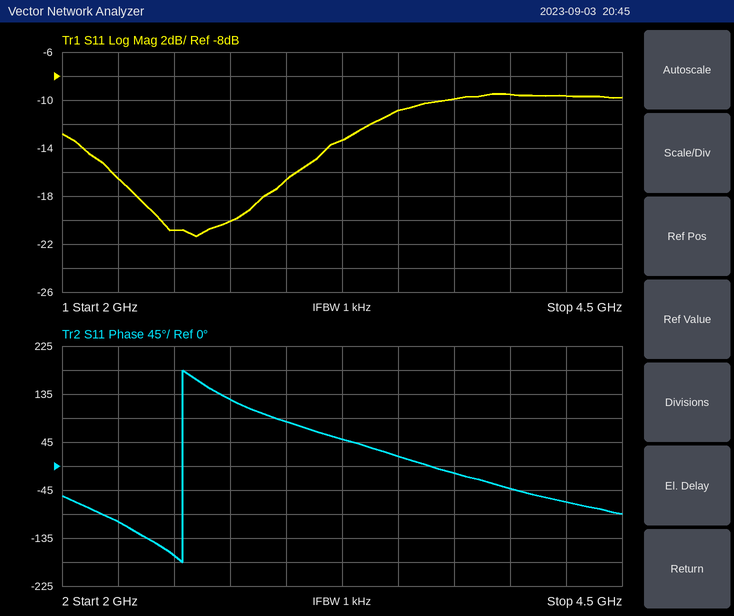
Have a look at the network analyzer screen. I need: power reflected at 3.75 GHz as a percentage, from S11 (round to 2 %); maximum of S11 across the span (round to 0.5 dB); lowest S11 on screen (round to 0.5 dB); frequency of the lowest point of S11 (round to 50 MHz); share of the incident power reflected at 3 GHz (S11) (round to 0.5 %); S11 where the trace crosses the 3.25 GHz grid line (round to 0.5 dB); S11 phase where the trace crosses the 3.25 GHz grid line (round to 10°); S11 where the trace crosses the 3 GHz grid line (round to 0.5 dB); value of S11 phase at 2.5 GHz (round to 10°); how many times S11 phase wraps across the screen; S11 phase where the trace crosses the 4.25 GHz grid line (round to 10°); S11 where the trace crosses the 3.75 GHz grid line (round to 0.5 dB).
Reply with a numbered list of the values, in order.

1. 10 %
2. -9.5 dB
3. -21.5 dB
4. 2.60 GHz
5. 2.0 %
6. -13.5 dB
7. 50°
8. -16.5 dB
9. -170°
10. 1
11. -70°
12. -10.0 dB
